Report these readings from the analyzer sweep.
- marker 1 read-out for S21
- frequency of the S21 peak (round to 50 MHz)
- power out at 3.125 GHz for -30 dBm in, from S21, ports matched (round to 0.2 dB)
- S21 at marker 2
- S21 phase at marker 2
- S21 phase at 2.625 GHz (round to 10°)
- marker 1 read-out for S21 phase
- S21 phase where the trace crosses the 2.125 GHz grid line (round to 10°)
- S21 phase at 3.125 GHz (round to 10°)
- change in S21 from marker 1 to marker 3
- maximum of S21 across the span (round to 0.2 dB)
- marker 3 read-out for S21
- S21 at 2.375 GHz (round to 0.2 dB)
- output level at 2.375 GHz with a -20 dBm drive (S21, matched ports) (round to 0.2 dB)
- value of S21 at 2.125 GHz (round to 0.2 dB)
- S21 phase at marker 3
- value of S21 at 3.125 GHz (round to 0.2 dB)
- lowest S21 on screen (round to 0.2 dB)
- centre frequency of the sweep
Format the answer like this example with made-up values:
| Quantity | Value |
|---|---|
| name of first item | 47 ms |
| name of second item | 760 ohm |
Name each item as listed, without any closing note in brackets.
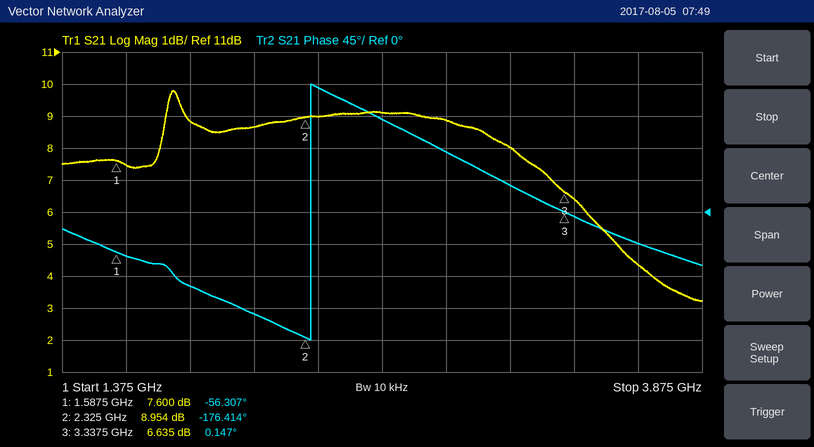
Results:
| Quantity | Value |
|---|---|
| marker 1 read-out for S21 | 7.600 dB |
| frequency of the S21 peak | 1.80 GHz |
| power out at 3.125 GHz for -30 dBm in, from S21, ports matched | -22.0 dBm |
| S21 at marker 2 | 8.954 dB |
| S21 phase at marker 2 | -176.414° |
| S21 phase at 2.625 GHz | 130° |
| marker 1 read-out for S21 phase | -56.307° |
| S21 phase where the trace crosses the 2.125 GHz grid line | -140° |
| S21 phase at 3.125 GHz | 40° |
| change in S21 from marker 1 to marker 3 | -0.965 dB |
| maximum of S21 across the span | 9.8 dB |
| marker 3 read-out for S21 | 6.635 dB |
| S21 at 2.375 GHz | 9.0 dB |
| output level at 2.375 GHz with a -20 dBm drive (S21, matched ports) | -11.0 dBm |
| value of S21 at 2.125 GHz | 8.6 dB |
| S21 phase at marker 3 | 0.147° |
| value of S21 at 3.125 GHz | 8.0 dB |
| lowest S21 on screen | 3.2 dB |
| centre frequency of the sweep | 2.625 GHz |
